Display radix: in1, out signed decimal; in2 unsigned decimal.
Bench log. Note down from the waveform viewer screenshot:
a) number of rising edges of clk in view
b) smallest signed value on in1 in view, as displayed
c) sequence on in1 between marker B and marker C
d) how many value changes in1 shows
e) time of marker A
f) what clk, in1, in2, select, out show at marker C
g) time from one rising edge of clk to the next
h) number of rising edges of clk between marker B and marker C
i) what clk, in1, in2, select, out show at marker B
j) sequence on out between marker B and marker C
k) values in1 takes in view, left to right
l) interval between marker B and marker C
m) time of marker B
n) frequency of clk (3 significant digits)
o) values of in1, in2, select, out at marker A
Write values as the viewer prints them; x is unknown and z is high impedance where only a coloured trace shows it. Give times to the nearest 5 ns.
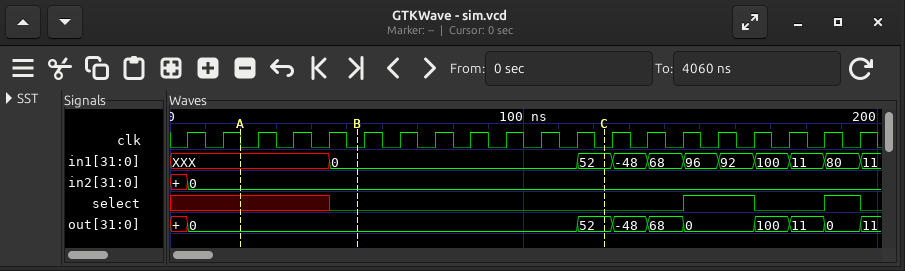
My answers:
20
-48
0, 52
10
20 ns
clk=0, in1=52, in2=0, select=0, out=52
10 ns
7
clk=0, in1=0, in2=0, select=0, out=0
0, 52
XXX, 0, 52, -48, 68, 96, 92, 100, 11, 80, 11
70 ns
55 ns
100 MHz
in1=XXX, in2=0, select=x, out=0
